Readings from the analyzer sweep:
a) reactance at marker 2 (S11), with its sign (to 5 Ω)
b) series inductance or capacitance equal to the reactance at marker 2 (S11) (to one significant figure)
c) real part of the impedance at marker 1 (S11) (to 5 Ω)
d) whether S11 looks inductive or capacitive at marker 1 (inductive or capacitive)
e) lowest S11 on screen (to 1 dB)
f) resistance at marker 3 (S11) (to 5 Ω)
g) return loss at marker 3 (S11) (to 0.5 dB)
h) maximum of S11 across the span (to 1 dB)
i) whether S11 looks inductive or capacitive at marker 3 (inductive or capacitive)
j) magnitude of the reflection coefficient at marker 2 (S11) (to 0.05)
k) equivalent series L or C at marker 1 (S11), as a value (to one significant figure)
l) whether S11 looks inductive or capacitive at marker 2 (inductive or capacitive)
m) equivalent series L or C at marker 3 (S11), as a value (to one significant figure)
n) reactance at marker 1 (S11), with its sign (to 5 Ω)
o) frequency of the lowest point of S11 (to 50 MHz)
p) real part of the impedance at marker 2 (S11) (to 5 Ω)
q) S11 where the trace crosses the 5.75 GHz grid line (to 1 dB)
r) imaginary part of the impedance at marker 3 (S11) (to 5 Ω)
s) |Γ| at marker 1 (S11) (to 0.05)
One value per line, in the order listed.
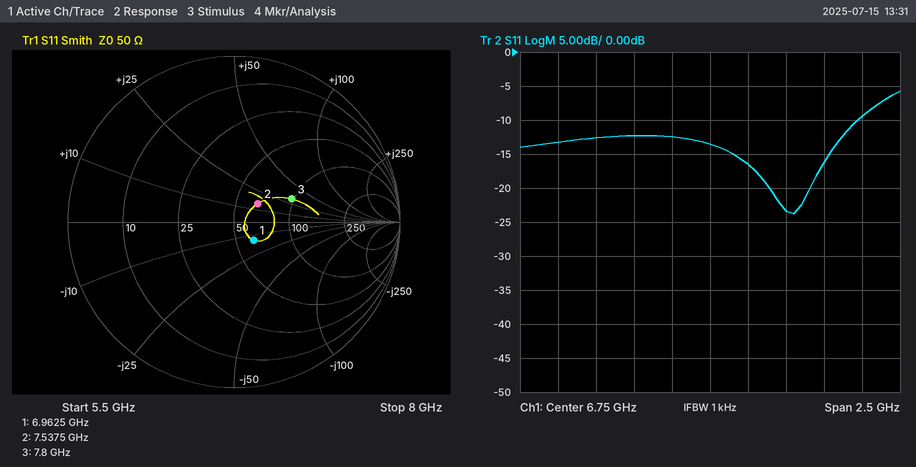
+15 Ω
300 pH
60 Ω
capacitive
-24 dB
95 Ω
8.5 dB
-6 dB
inductive
0.20
2 pF
inductive
600 pH
-15 Ω
7.30 GHz
65 Ω
-13 dB
+30 Ω
0.15
